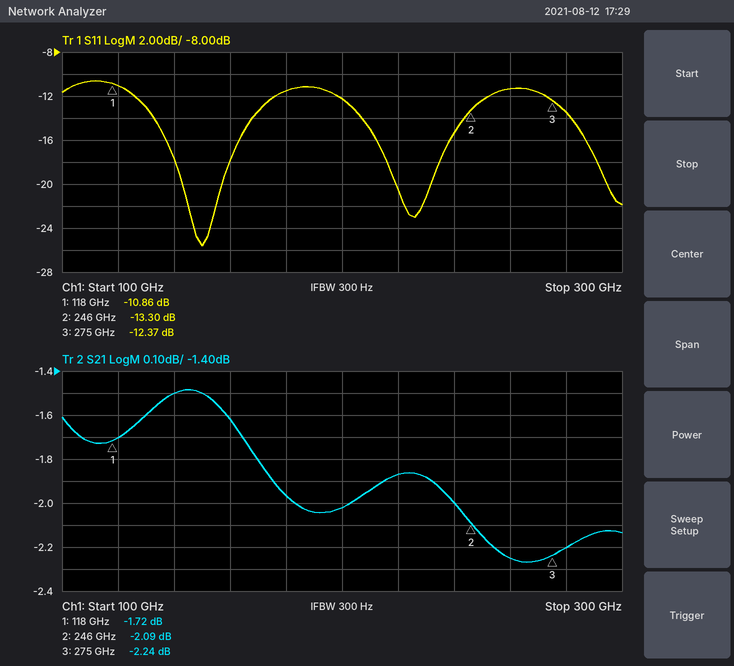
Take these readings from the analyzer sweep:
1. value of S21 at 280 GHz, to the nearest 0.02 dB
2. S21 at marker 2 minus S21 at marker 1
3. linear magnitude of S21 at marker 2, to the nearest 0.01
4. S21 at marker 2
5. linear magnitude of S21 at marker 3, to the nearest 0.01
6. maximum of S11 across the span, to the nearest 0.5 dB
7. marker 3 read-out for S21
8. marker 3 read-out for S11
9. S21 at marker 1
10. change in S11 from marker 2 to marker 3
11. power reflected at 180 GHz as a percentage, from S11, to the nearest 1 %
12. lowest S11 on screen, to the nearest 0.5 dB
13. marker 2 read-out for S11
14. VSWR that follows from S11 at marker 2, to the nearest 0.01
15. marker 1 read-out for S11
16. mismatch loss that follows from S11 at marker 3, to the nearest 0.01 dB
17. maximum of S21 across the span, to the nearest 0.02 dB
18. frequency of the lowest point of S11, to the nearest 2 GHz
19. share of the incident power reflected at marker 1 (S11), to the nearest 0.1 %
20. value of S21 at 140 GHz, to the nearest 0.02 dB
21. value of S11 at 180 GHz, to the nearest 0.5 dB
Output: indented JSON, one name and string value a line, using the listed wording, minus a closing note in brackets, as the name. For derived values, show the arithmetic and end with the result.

{
  "value of S21 at 280 GHz, to the nearest 0.02 dB": "-2.20 dB",
  "S21 at marker 2 minus S21 at marker 1": "-2.09 − (-1.72) = -0.37 dB",
  "linear magnitude of S21 at marker 2, to the nearest 0.01": "10^(-2.09/20) ≈ 0.79",
  "S21 at marker 2": "-2.09 dB",
  "linear magnitude of S21 at marker 3, to the nearest 0.01": "10^(-2.24/20) ≈ 0.77",
  "maximum of S11 across the span, to the nearest 0.5 dB": "-10.5 dB",
  "marker 3 read-out for S21": "-2.24 dB",
  "marker 3 read-out for S11": "-12.37 dB",
  "S21 at marker 1": "-1.72 dB",
  "change in S11 from marker 2 to marker 3": "-12.37 − (-13.3) = 0.93 dB",
  "power reflected at 180 GHz as a percentage, from S11, to the nearest 1 %": "10^(-11.5/10) ≈ 7 %",
  "lowest S11 on screen, to the nearest 0.5 dB": "-25.5 dB",
  "marker 2 read-out for S11": "-13.30 dB",
  "VSWR that follows from S11 at marker 2, to the nearest 0.01": "(1 + 0.2163)/(1 − 0.2163) ≈ 1.55",
  "marker 1 read-out for S11": "-10.86 dB",
  "mismatch loss that follows from S11 at marker 3, to the nearest 0.01 dB": "−10 log10(1 − 10^(-12.37/10)) ≈ 0.26 dB",
  "maximum of S21 across the span, to the nearest 0.02 dB": "-1.48 dB",
  "frequency of the lowest point of S11, to the nearest 2 GHz": "150 GHz",
  "share of the incident power reflected at marker 1 (S11), to the nearest 0.1 %": "10^(-10.86/10) ≈ 8.2 %",
  "value of S21 at 140 GHz, to the nearest 0.02 dB": "-1.50 dB",
  "value of S11 at 180 GHz, to the nearest 0.5 dB": "-11.5 dB"
}
